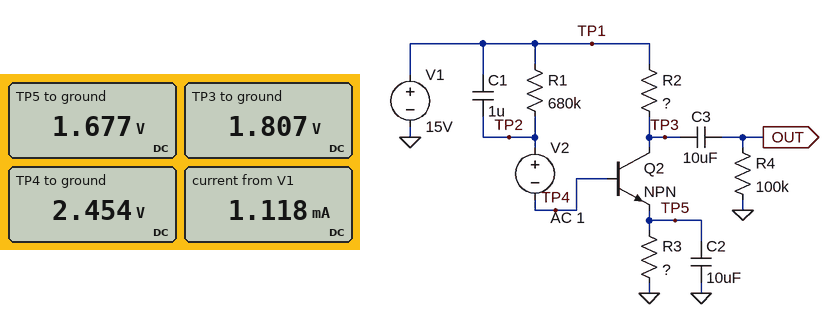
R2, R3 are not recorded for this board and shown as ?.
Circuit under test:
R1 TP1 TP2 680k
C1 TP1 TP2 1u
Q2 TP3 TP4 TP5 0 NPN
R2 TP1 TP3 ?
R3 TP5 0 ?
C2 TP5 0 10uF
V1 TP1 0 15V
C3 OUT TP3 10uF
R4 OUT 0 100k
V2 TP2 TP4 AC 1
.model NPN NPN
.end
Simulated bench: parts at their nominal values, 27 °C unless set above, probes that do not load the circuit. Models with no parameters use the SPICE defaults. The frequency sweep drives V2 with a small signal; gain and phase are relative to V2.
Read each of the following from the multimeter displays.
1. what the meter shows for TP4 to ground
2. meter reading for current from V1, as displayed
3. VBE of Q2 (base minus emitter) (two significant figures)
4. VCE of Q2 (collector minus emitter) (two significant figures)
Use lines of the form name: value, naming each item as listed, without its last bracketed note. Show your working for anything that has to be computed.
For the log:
what the meter shows for TP4 to ground: 2.454 V
meter reading for current from V1, as displayed: 1.118 mA
VBE of Q2 (base minus emitter): 2.454 V - 1.677 V = 780 mV
VCE of Q2 (collector minus emitter): 1.807 V - 1.677 V = 130 mV
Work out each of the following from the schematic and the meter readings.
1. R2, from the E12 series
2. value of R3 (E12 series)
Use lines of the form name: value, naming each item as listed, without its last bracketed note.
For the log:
R2, from the E12 series: 12 kΩ
value of R3: 1.5 kΩ
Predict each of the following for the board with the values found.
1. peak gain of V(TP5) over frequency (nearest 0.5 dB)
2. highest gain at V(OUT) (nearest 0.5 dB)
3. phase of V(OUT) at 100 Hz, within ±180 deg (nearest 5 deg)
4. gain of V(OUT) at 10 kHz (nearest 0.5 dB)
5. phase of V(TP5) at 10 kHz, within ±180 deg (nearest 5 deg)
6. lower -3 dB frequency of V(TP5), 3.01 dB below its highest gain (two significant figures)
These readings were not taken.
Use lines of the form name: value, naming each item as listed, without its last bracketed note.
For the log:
peak gain of V(TP5) over frequency: -18.5 dB
highest gain at V(OUT): 36.0 dB
phase of V(OUT) at 100 Hz, within ±180 deg: 90 deg
gain of V(OUT) at 10 kHz: 35.5 dB
phase of V(TP5) at 10 kHz, within ±180 deg: 110 deg
lower -3 dB frequency of V(TP5), 3.01 dB below its highest gain: 11 Hz
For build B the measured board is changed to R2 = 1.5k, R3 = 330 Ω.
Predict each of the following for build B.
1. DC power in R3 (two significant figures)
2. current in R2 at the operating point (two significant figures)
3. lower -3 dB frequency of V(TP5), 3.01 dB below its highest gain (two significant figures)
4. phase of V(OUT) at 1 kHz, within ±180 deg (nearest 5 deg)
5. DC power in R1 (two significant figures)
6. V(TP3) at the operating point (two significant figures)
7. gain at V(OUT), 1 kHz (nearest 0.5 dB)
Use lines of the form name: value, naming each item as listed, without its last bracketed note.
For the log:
DC power in R3: 1.3 mW
current in R2 at the operating point: 2.0 mA
lower -3 dB frequency of V(TP5), 3.01 dB below its highest gain: 4.4 Hz
phase of V(OUT) at 1 kHz, within ±180 deg: 50 deg
DC power in R1: 270 µW
V(TP3) at the operating point: 12 V
gain at V(OUT), 1 kHz: 36.5 dB
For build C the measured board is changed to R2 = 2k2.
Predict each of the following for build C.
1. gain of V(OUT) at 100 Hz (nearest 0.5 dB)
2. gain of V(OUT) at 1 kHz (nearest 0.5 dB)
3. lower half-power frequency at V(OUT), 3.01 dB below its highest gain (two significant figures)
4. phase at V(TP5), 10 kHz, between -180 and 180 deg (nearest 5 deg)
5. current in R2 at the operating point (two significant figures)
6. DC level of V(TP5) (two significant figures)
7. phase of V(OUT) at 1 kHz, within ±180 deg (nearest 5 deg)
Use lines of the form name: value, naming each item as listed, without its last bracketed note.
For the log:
gain of V(OUT) at 100 Hz: 21.5 dB
gain of V(OUT) at 1 kHz: 39.5 dB
lower half-power frequency at V(OUT), 3.01 dB below its highest gain: 1.2 kHz
phase at V(TP5), 10 kHz, between -180 and 180 deg: 95 deg
current in R2 at the operating point: 1.7 mA
DC level of V(TP5): 2.6 V
phase of V(OUT) at 1 kHz, within ±180 deg: 50 deg
